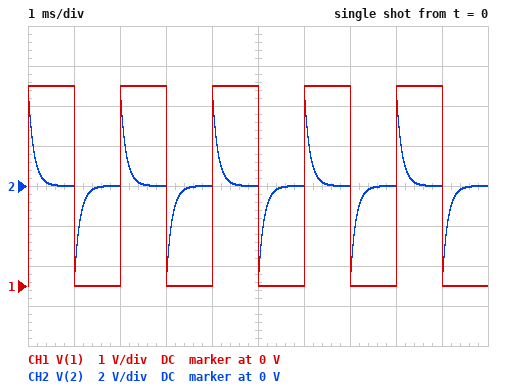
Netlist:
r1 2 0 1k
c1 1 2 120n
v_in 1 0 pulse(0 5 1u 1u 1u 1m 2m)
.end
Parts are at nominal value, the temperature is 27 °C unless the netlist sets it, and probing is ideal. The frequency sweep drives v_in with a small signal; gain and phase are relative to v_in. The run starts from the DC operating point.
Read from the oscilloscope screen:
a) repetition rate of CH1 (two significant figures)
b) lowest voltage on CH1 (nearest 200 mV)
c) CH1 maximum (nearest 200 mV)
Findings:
500 Hz
0 V
5.0 V
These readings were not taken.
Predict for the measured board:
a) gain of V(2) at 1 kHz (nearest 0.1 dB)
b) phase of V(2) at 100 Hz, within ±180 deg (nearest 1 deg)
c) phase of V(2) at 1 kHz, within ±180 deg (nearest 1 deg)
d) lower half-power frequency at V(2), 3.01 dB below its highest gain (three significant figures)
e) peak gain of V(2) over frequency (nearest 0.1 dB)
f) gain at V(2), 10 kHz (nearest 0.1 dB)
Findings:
-4.4 dB
86 deg
53 deg
1.33 kHz
0 dB
-0.1 dB
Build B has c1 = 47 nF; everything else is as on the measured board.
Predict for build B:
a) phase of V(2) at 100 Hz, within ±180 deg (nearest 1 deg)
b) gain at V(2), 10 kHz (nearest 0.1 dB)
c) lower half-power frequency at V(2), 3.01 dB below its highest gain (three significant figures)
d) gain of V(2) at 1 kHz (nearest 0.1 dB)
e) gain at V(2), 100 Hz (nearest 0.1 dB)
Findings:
88 deg
-0.5 dB
3.39 kHz
-11.0 dB
-30.6 dB
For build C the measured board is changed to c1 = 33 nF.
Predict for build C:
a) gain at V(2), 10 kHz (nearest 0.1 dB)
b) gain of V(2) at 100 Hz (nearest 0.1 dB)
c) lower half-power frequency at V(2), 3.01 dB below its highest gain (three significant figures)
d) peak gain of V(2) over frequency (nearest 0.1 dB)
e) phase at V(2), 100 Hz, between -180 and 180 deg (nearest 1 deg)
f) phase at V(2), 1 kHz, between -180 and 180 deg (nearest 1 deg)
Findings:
-0.9 dB
-33.7 dB
4.82 kHz
0 dB
89 deg
78 deg
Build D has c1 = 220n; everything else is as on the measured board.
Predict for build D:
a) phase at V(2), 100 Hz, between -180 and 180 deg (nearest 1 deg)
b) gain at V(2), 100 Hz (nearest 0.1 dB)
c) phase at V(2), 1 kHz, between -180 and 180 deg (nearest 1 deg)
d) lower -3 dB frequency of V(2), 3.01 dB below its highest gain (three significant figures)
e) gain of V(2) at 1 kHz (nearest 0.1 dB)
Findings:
82 deg
-17.3 dB
36 deg
723 Hz
-1.8 dB
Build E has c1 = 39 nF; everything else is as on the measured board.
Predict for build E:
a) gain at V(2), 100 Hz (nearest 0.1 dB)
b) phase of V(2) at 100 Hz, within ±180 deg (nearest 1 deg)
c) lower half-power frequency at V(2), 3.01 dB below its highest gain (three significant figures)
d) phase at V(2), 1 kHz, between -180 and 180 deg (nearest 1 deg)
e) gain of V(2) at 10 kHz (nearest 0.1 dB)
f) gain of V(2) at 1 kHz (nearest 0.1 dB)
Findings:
-32.2 dB
89 deg
4.08 kHz
76 deg
-0.7 dB
-12.5 dB
